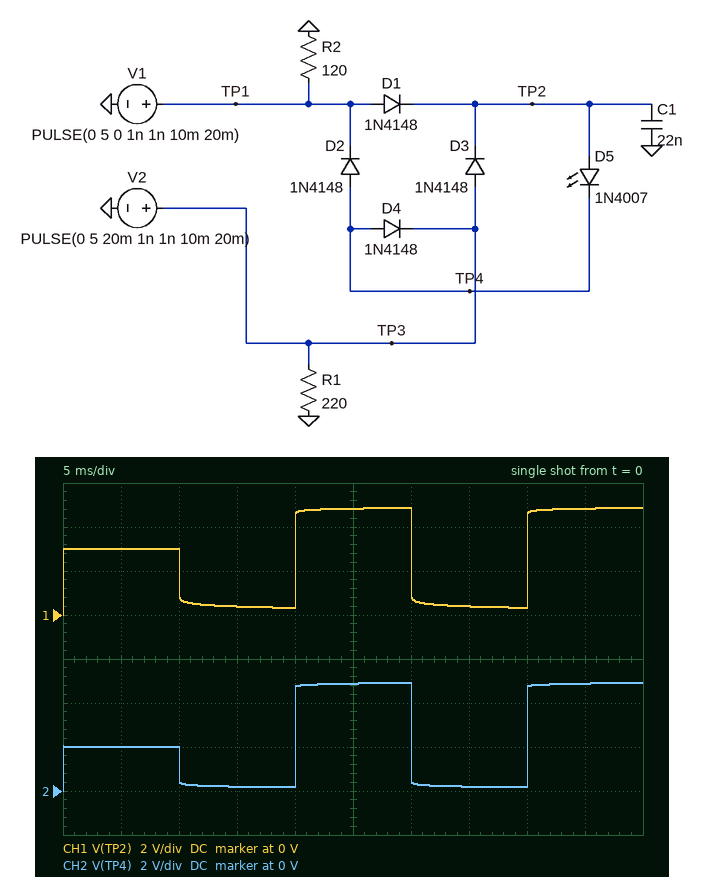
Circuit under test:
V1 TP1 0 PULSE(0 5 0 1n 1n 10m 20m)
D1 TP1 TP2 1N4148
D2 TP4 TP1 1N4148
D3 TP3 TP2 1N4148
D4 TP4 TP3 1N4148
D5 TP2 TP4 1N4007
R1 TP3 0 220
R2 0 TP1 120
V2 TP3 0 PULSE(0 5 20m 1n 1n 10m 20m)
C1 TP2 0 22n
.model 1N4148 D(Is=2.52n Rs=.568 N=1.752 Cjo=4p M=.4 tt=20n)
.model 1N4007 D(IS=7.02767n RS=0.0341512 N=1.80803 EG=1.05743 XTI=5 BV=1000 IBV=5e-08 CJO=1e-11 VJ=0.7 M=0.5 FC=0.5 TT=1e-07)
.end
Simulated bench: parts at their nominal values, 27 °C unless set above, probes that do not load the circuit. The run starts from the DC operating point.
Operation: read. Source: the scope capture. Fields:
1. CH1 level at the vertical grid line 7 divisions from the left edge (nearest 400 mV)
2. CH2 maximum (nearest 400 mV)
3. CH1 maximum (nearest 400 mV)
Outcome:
400 mV
4.8 V
4.8 V
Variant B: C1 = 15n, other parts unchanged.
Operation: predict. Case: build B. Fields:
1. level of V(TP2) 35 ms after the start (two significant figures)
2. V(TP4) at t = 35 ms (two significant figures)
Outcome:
350 mV
180 mV
